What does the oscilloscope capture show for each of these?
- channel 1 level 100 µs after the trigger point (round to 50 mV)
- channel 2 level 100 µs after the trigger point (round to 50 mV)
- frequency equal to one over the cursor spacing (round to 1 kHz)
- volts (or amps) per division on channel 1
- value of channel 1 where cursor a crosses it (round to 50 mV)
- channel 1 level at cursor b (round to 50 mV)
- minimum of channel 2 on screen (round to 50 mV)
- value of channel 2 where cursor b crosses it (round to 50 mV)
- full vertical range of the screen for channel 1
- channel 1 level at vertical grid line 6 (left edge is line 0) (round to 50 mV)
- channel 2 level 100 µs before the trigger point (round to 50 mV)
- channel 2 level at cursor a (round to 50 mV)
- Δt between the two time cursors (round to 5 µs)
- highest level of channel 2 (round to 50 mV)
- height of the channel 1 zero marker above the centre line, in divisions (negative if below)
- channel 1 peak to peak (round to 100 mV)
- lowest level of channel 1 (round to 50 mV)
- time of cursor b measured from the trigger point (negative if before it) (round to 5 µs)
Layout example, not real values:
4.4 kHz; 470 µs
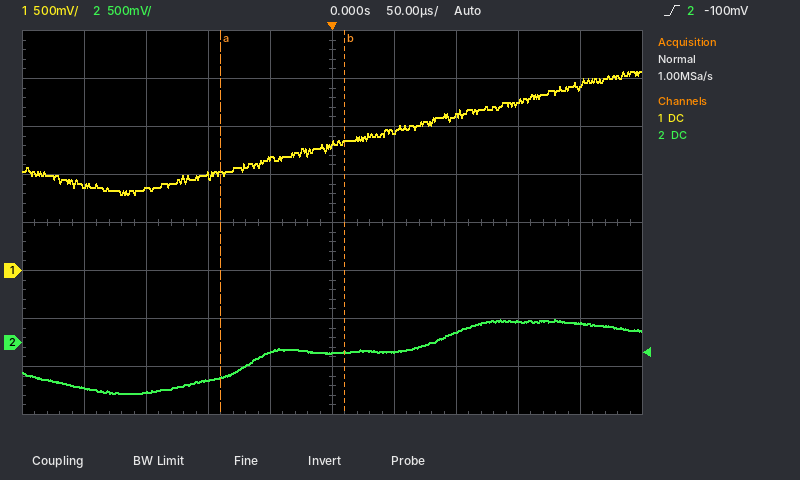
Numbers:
1.60 V; 100 mV; 10 kHz; 500 mV; 1.00 V; 1.35 V; -550 mV; -100 mV; 4 V; 1.45 V; -400 mV; -350 mV; 100 µs; 250 mV; -1.0 div; 1.30 V; 800 mV; +10 µs
